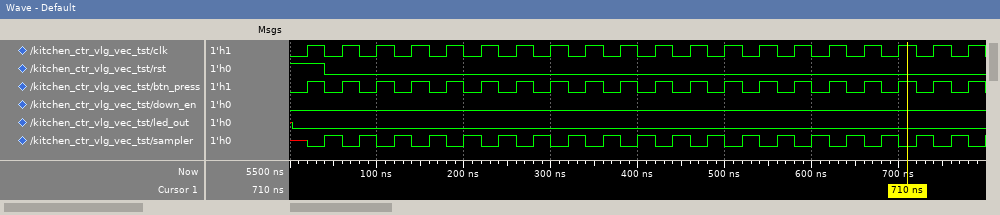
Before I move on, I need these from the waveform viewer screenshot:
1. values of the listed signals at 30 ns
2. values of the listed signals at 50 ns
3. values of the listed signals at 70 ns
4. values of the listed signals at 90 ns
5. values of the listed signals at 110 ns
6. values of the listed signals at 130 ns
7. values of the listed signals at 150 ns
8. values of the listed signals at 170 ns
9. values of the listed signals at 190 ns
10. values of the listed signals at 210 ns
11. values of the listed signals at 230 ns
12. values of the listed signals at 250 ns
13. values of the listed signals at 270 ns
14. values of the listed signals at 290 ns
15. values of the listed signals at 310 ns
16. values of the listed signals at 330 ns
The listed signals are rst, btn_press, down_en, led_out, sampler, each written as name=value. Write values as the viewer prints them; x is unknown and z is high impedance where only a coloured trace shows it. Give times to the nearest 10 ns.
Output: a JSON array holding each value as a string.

["rst=1, btn_press=1, down_en=0, led_out=0, sampler=0", "rst=0, btn_press=0, down_en=0, led_out=0, sampler=1", "rst=0, btn_press=1, down_en=0, led_out=0, sampler=0", "rst=0, btn_press=0, down_en=0, led_out=0, sampler=1", "rst=0, btn_press=1, down_en=0, led_out=0, sampler=0", "rst=0, btn_press=0, down_en=0, led_out=0, sampler=1", "rst=0, btn_press=1, down_en=0, led_out=0, sampler=0", "rst=0, btn_press=0, down_en=0, led_out=0, sampler=1", "rst=0, btn_press=1, down_en=0, led_out=0, sampler=0", "rst=0, btn_press=0, down_en=0, led_out=0, sampler=1", "rst=0, btn_press=1, down_en=0, led_out=0, sampler=0", "rst=0, btn_press=0, down_en=0, led_out=0, sampler=1", "rst=0, btn_press=1, down_en=0, led_out=0, sampler=0", "rst=0, btn_press=0, down_en=0, led_out=0, sampler=1", "rst=0, btn_press=1, down_en=0, led_out=0, sampler=0", "rst=0, btn_press=0, down_en=0, led_out=0, sampler=1"]
